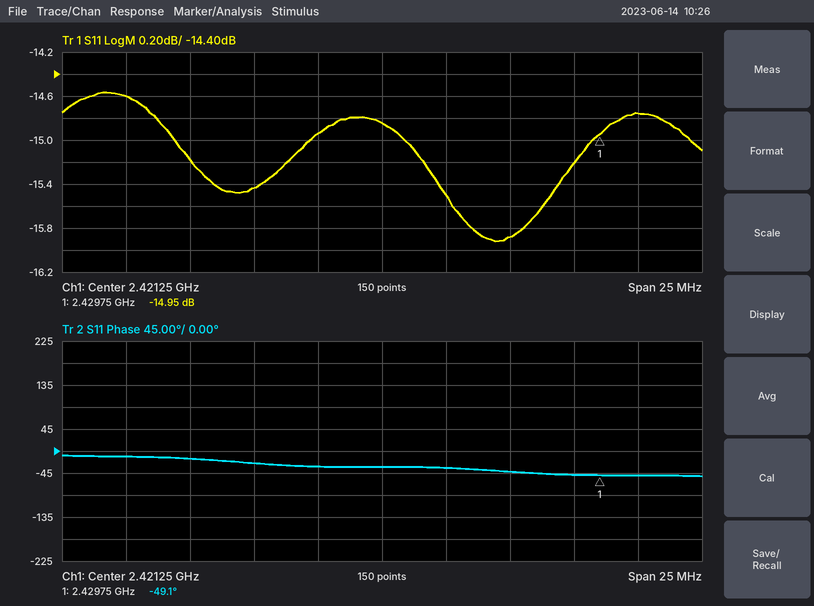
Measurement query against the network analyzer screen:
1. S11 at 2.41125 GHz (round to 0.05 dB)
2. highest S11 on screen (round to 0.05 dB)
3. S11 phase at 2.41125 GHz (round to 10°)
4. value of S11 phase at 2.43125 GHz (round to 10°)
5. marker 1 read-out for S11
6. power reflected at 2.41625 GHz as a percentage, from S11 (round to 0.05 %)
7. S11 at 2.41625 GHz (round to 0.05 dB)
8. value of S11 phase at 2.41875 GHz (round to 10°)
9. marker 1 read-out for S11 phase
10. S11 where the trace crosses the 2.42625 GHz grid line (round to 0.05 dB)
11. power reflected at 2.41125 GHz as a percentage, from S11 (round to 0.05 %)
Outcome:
-14.60 dB
-14.55 dB
-10°
-50°
-14.95 dB
2.85 %
-15.45 dB
-30°
-49.1°
-15.90 dB
3.45 %
